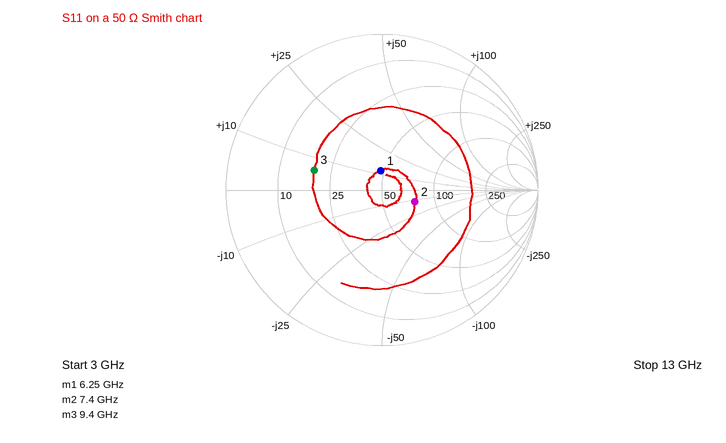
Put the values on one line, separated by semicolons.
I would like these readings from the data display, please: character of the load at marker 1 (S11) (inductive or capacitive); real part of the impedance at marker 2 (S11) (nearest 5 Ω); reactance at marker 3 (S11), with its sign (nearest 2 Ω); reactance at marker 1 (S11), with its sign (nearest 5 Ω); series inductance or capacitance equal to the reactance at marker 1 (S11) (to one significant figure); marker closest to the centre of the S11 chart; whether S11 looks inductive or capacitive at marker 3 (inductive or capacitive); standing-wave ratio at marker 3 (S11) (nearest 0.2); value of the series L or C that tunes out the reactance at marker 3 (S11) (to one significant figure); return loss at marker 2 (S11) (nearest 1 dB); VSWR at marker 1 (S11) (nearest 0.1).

inductive; 75 Ω; +6 Ω; +10 Ω; 300 pH; marker 1; inductive; 2.6; 3 pF; 13 dB; 1.3
